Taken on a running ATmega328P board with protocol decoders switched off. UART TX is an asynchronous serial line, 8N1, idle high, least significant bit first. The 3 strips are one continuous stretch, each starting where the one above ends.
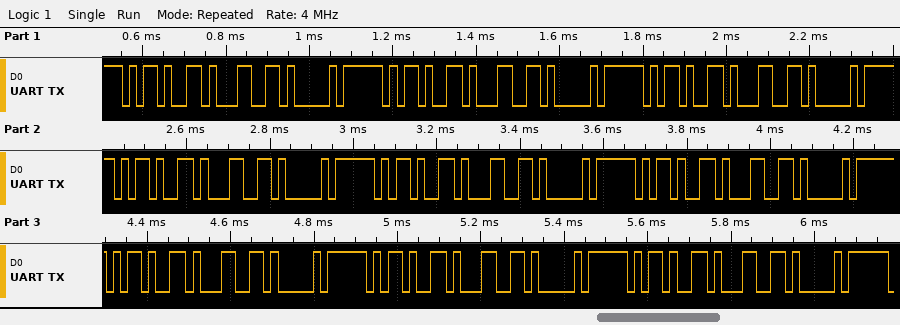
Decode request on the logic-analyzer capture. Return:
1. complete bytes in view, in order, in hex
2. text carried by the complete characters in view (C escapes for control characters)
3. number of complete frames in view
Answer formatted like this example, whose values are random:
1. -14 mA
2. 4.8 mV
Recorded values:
1. 2D 31 41 2D 31 41 2D 31 41 2D 31 41 2D 31 41 2D 31 41 2D 31 41 2D 31 41 2D 31 41
2. "-1A-1A-1A-1A-1A-1A-1A-1A-1A"
3. 27
